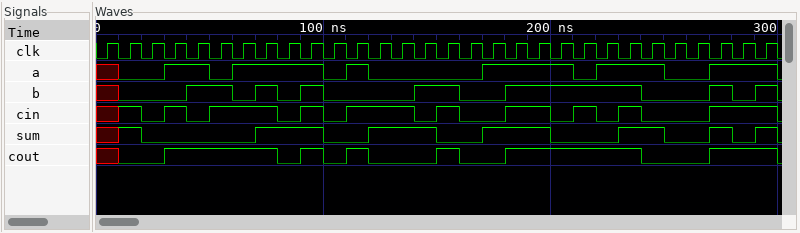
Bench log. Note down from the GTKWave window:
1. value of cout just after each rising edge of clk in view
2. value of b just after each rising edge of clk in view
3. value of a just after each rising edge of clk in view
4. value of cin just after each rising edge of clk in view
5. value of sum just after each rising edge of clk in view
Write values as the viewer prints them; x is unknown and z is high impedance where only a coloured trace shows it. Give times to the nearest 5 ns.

x 0 0 1 1 1 1 1 0 1 0 1 0 0 0 1 0 0 1 1 1 1 1 1 0 0 0 1 1 1
x 0 0 0 1 1 0 1 0 1 0 0 0 0 1 1 0 0 1 1 1 1 1 1 0 0 0 1 0 1
x 0 0 1 1 0 1 1 1 1 0 1 0 0 0 0 0 1 1 1 1 0 1 1 1 0 0 1 1 1
x 1 0 1 0 1 1 1 0 1 0 1 1 1 0 1 0 0 1 1 0 1 0 1 0 0 0 1 1 1
x 1 0 0 0 0 0 1 1 1 0 0 1 1 1 0 0 1 1 1 0 0 0 1 1 0 0 1 0 1
